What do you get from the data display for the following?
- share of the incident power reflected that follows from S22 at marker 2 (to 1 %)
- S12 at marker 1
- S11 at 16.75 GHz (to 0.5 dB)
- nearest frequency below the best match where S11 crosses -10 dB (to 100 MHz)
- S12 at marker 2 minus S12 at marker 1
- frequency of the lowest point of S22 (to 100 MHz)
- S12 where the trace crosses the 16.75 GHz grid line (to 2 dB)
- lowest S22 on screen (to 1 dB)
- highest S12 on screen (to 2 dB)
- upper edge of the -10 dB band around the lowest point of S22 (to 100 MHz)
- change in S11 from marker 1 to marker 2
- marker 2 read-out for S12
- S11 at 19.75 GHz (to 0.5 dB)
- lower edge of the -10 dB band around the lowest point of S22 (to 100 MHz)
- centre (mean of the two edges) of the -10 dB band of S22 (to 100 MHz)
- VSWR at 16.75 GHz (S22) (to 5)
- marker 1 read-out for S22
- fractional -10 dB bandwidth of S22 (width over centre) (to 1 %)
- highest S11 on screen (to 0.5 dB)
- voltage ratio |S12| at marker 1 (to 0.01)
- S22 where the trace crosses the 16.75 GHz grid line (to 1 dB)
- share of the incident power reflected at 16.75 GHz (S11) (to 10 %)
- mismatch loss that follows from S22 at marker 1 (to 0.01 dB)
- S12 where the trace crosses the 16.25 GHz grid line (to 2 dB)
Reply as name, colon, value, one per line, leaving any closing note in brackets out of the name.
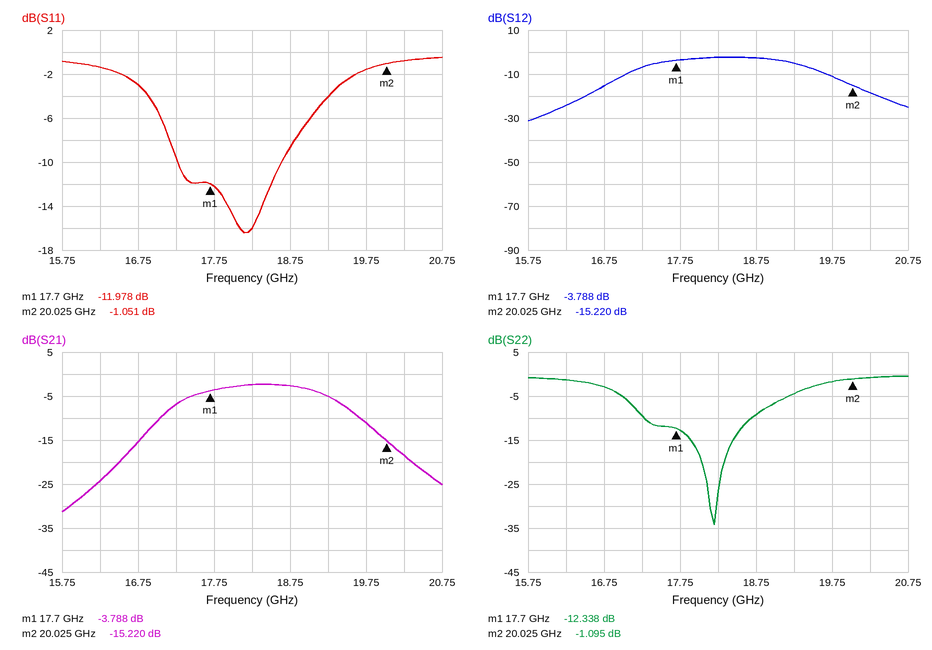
share of the incident power reflected that follows from S22 at marker 2: 78 %
S12 at marker 1: -3.788 dB
S11 at 16.75 GHz: -3.0 dB
nearest frequency below the best match where S11 crosses -10 dB: 17.3 GHz
S12 at marker 2 minus S12 at marker 1: -11.432 dB
frequency of the lowest point of S22: 18.2 GHz
S12 where the trace crosses the 16.75 GHz grid line: -16 dB
lowest S22 on screen: -34 dB
highest S12 on screen: -2 dB
upper edge of the -10 dB band around the lowest point of S22: 18.7 GHz
change in S11 from marker 1 to marker 2: 10.927 dB
marker 2 read-out for S12: -15.220 dB
S11 at 19.75 GHz: -1.5 dB
lower edge of the -10 dB band around the lowest point of S22: 17.3 GHz
centre (mean of the two edges) of the -10 dB band of S22: 18.0 GHz
VSWR at 16.75 GHz (S22): 5
marker 1 read-out for S22: -12.338 dB
fractional -10 dB bandwidth of S22 (width over centre): 8 %
highest S11 on screen: -0.5 dB
voltage ratio |S12| at marker 1: 0.65
S22 where the trace crosses the 16.75 GHz grid line: -3 dB
share of the incident power reflected at 16.75 GHz (S11): 50 %
mismatch loss that follows from S22 at marker 1: 0.26 dB
S12 where the trace crosses the 16.25 GHz grid line: -24 dB
